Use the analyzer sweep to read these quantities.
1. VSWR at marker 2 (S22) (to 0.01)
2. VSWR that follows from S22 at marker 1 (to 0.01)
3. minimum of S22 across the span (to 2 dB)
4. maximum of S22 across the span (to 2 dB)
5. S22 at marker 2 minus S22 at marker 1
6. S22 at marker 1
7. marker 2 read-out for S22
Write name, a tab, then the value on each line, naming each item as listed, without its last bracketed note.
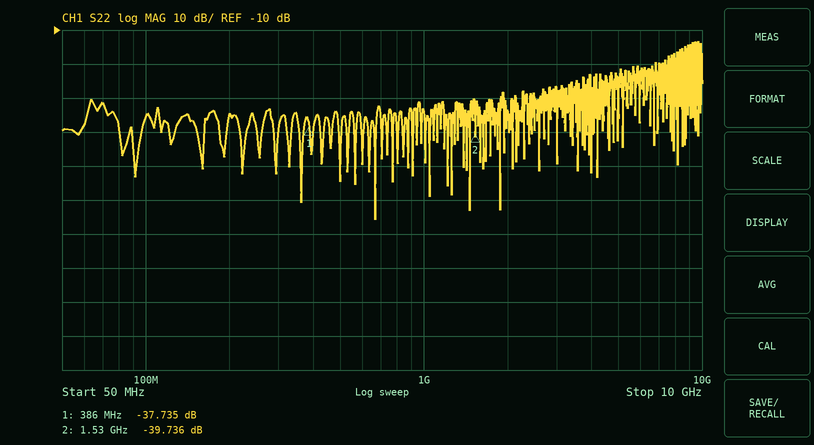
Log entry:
VSWR at marker 2 (S22)	1.02
VSWR that follows from S22 at marker 1	1.03
minimum of S22 across the span	-66 dB
maximum of S22 across the span	-14 dB
S22 at marker 2 minus S22 at marker 1	-2.001 dB
S22 at marker 1	-37.735 dB
marker 2 read-out for S22	-39.736 dB
